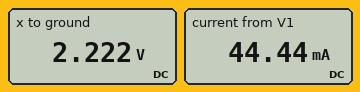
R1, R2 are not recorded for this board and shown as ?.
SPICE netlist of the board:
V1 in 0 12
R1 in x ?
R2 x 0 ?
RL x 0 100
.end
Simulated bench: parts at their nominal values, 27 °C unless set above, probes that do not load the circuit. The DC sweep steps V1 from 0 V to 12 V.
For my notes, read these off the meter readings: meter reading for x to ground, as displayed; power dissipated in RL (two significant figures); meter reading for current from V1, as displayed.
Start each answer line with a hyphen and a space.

- 2.222 V
- 49 mW
- 44.44 mA
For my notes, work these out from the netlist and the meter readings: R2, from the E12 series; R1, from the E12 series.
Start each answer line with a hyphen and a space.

- 100 Ω
- 220 Ω
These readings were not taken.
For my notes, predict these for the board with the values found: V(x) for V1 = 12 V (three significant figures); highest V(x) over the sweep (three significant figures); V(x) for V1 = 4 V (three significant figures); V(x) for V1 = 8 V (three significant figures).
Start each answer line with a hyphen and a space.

- 2.22 V
- 2.22 V
- 741 mV
- 1.48 V
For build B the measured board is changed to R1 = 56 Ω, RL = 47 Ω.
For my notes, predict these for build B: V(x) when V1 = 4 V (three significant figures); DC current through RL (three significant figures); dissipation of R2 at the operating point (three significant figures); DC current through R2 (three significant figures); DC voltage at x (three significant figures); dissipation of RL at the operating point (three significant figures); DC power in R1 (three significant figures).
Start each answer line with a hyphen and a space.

- 1.45 V
- 92.8 mA
- 190 mW
- 43.6 mA
- 4.36 V
- 405 mW
- 1.04 W
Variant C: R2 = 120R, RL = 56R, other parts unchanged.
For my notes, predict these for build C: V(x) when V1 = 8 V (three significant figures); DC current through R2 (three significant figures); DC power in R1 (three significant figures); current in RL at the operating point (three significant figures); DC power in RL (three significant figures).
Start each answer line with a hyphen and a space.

- 1.18 V
- 14.8 mA
- 475 mW
- 31.7 mA
- 56.2 mW
